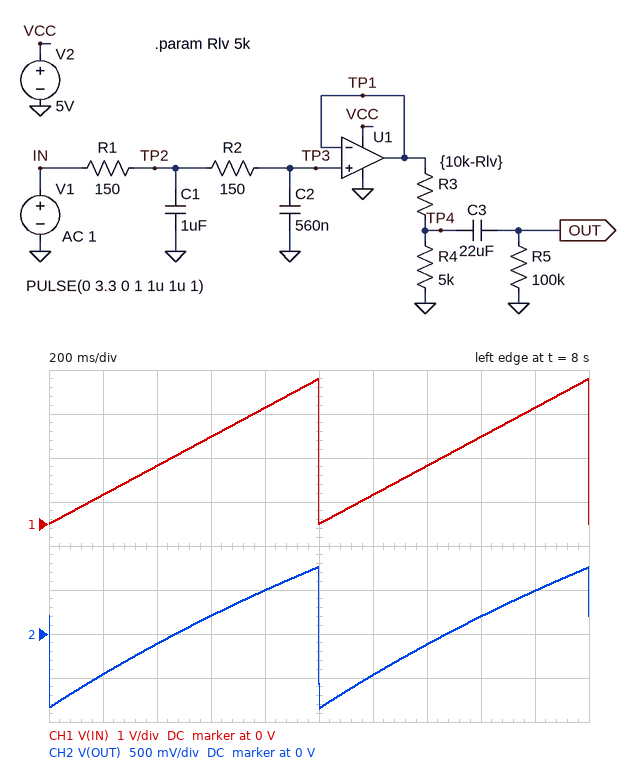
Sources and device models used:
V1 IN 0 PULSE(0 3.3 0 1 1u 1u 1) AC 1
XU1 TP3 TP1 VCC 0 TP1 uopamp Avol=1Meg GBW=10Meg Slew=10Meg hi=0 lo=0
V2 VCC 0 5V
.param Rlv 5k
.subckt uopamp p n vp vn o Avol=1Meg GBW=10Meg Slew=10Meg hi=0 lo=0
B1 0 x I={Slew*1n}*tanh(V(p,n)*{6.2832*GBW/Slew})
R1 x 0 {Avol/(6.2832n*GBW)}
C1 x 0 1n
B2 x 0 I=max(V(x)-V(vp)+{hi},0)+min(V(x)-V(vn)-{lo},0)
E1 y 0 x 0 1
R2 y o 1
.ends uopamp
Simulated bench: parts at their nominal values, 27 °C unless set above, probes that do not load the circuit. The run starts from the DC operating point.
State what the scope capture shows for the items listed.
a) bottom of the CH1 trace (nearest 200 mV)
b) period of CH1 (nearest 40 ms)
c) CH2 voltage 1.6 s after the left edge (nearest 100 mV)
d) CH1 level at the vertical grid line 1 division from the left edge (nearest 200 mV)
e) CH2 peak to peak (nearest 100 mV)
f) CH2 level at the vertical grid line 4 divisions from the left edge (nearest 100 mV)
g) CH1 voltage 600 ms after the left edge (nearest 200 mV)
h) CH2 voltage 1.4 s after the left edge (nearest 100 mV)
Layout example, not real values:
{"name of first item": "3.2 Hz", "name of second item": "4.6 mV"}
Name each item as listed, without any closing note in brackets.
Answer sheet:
{"bottom of the CH1 trace": "0 V", "period of CH1": "1.00 s", "CH2 voltage 1.6 s after the left edge": "200 mV", "CH1 level at the vertical grid line 1 division from the left edge": "600 mV", "CH2 peak to peak": "1.6 V", "CH2 level at the vertical grid line 4 divisions from the left edge": "500 mV", "CH1 voltage 600 ms after the left edge": "2.0 V", "CH2 voltage 1.4 s after the left edge": "-100 mV"}
